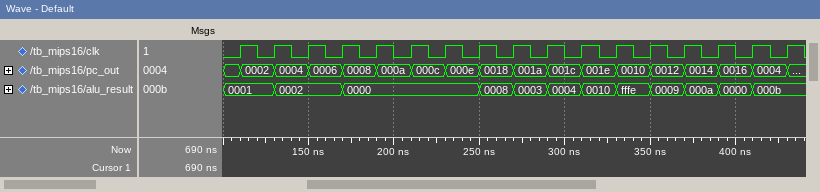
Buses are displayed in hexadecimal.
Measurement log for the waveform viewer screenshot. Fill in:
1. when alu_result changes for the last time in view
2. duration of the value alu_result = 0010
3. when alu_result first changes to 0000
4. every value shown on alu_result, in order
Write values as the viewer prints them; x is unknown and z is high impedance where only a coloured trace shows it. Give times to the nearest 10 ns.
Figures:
410 ns
20 ns
170 ns
0001, 0002, 0000, 0008, 0003, 0004, 0010, fffe, 0009, 000a, 0000, 000b
